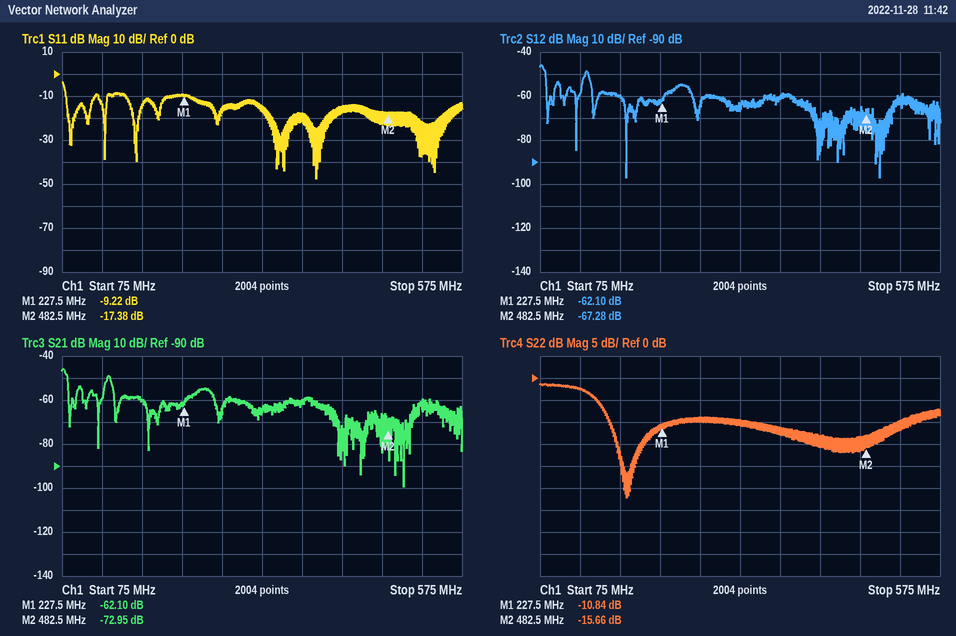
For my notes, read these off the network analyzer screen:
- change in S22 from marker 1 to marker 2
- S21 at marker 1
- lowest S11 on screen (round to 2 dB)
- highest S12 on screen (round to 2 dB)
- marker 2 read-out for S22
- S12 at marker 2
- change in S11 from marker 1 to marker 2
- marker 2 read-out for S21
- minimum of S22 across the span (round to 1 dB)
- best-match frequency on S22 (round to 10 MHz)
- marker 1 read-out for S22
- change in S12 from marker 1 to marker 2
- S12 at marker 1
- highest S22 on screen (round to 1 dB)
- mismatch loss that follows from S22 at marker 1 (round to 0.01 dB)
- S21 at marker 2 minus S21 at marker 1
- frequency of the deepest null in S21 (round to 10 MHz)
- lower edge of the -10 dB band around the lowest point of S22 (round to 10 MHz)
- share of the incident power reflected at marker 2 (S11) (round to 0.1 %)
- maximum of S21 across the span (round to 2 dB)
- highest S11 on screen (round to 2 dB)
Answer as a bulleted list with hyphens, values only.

- -4.82 dB
- -62.10 dB
- -48 dB
- -46 dB
- -15.66 dB
- -67.28 dB
- -8.16 dB
- -72.95 dB
- -27 dB
- 180 MHz
- -10.84 dB
- -5.18 dB
- -62.10 dB
- -1 dB
- 0.37 dB
- -10.85 dB
- 500 MHz
- 160 MHz
- 1.8 %
- -46 dB
- -4 dB
